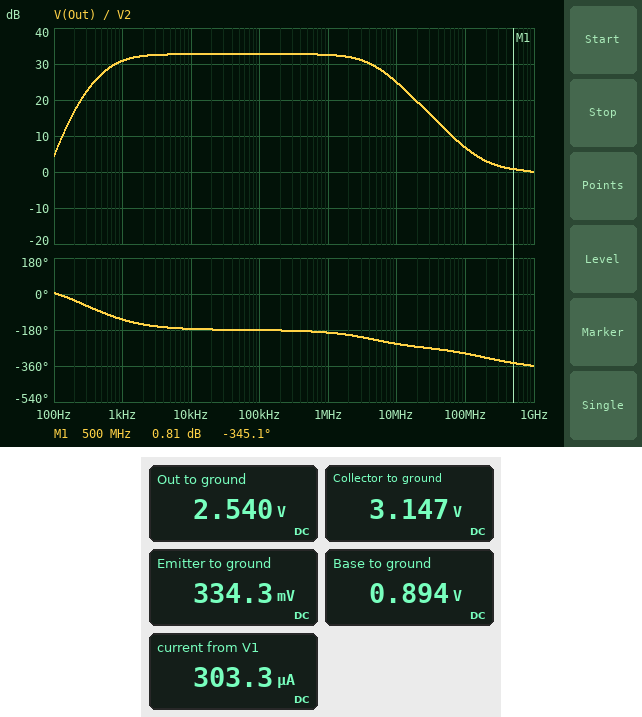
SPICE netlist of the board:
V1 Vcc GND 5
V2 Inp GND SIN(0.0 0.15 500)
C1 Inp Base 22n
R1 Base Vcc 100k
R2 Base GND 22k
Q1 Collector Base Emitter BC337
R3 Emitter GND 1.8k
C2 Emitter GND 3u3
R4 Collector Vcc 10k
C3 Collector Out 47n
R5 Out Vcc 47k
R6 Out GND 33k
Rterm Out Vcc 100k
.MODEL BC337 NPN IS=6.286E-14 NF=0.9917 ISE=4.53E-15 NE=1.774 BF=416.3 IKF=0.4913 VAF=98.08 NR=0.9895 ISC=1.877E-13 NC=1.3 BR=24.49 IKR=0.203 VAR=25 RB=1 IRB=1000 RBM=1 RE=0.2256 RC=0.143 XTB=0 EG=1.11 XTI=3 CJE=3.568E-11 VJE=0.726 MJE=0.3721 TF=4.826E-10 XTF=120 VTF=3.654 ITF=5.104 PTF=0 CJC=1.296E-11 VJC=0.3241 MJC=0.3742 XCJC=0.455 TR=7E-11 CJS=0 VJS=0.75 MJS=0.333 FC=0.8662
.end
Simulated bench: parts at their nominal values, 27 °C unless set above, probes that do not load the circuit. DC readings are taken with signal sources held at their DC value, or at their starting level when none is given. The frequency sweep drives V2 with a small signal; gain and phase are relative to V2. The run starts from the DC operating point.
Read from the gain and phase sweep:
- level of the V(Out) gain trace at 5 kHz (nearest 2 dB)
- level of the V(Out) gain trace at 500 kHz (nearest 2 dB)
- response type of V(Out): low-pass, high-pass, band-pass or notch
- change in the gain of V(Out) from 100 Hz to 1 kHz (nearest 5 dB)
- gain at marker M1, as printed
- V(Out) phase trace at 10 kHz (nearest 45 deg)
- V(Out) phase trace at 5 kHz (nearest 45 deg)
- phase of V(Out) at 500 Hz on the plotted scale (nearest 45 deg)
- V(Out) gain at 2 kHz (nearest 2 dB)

32 dB
32 dB
band-pass
25 dB
0.81 dB
-180 deg
-180 deg
-90 deg
32 dB
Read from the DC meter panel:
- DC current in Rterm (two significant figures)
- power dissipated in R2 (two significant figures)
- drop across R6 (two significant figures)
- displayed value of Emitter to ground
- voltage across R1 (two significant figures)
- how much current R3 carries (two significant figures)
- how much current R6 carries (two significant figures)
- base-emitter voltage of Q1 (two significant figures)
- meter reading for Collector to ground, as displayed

25 µA
36 µW
2.5 V
334.3 mV
4.1 V
190 µA
77 µA
560 mV
3.147 V
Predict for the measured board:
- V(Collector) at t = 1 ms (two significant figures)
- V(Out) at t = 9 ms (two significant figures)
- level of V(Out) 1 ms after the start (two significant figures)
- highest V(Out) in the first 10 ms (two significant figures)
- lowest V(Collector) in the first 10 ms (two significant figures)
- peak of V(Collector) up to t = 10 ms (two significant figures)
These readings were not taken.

4.2 V
3.8 V
3.8 V
4.0 V
400 mV
4.4 V
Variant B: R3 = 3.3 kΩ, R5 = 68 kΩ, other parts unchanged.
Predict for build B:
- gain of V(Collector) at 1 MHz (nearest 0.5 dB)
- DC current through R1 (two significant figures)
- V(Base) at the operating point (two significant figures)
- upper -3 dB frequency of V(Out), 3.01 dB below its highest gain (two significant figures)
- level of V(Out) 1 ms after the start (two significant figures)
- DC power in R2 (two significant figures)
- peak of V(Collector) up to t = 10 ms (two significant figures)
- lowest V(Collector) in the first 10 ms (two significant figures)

28.0 dB
41 µA
900 mV
4.6 MHz
3.2 V
37 µW
4.7 V
480 mV
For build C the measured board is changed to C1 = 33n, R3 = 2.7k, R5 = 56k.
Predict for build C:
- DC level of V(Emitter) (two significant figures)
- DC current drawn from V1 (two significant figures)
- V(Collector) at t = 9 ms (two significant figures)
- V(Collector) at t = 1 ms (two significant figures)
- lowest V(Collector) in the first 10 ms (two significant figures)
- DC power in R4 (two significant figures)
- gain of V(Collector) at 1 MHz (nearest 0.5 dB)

350 mV
240 µA
4.4 V
4.3 V
430 mV
160 µW
29.5 dB
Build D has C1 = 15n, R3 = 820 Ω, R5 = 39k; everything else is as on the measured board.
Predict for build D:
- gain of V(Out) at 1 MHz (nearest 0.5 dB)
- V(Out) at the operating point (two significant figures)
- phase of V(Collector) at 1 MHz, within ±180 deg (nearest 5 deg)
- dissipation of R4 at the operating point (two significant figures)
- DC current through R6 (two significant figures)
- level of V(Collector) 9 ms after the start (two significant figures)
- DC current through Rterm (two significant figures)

37.5 dB
2.7 V
160 deg
1.4 mW
82 µA
3.3 V
23 µA
